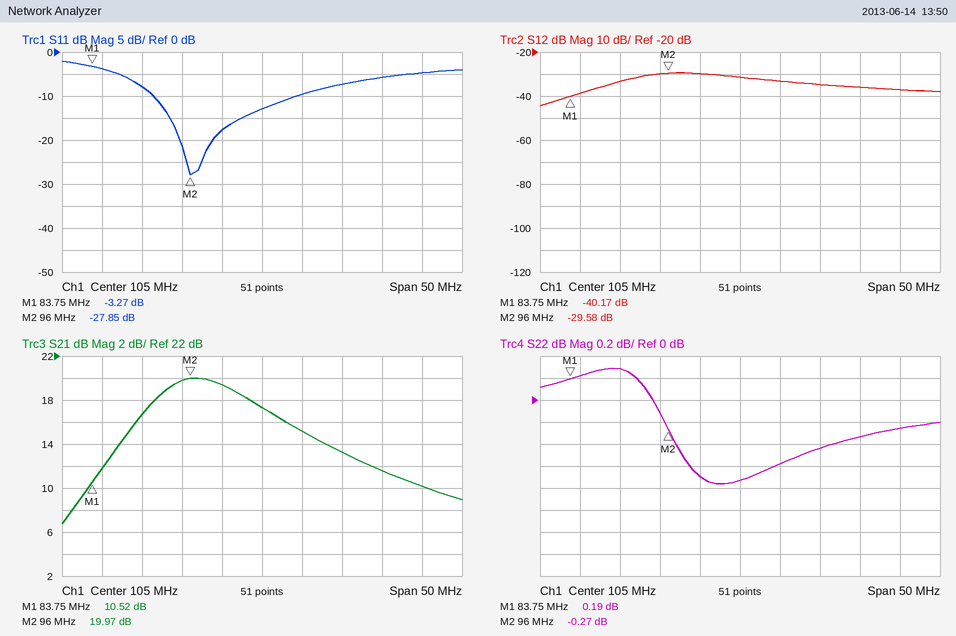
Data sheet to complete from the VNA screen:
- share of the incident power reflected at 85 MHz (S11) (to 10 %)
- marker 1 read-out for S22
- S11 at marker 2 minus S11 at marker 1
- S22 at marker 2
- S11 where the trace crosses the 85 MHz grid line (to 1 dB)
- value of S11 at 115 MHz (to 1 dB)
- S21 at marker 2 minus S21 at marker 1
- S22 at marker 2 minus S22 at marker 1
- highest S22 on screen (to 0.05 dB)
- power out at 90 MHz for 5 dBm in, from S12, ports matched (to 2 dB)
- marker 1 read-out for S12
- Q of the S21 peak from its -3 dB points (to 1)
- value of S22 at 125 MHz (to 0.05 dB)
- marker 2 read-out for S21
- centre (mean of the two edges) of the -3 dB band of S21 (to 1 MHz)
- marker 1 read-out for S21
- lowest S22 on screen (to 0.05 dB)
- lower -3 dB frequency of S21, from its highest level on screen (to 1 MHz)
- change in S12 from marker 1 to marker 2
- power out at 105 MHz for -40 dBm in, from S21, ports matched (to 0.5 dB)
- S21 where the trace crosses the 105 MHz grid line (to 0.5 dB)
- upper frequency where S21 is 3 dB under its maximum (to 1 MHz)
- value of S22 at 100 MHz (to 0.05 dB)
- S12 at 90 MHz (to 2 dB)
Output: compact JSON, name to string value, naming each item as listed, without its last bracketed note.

{"share of the incident power reflected at 85 MHz (S11)": "40 %", "marker 1 read-out for S22": "0.19 dB", "S11 at marker 2 minus S11 at marker 1": "-24.58 dB", "S22 at marker 2": "-0.27 dB", "S11 where the trace crosses the 85 MHz grid line": "-4 dB", "value of S11 at 115 MHz": "-7 dB", "S21 at marker 2 minus S21 at marker 1": "9.45 dB", "S22 at marker 2 minus S22 at marker 1": "-0.46 dB", "highest S22 on screen": "0.30 dB", "power out at 90 MHz for 5 dBm in, from S12, ports matched": "-28 dBm", "marker 1 read-out for S12": "-40.17 dB", "Q of the S21 peak from its -3 dB points": "6", "value of S22 at 125 MHz": "-0.25 dB", "marker 2 read-out for S21": "19.97 dB", "centre (mean of the two edges) of the -3 dB band of S21": "98 MHz", "marker 1 read-out for S21": "10.52 dB", "lowest S22 on screen": "-0.75 dB", "lower -3 dB frequency of S21, from its highest level on screen": "90 MHz", "change in S12 from marker 1 to marker 2": "10.59 dB", "power out at 105 MHz for -40 dBm in, from S21, ports matched": "-22.5 dBm", "S21 where the trace crosses the 105 MHz grid line": "17.5 dB", "upper frequency where S21 is 3 dB under its maximum": "106 MHz", "value of S22 at 100 MHz": "-0.70 dB", "S12 at 90 MHz": "-34 dB"}
